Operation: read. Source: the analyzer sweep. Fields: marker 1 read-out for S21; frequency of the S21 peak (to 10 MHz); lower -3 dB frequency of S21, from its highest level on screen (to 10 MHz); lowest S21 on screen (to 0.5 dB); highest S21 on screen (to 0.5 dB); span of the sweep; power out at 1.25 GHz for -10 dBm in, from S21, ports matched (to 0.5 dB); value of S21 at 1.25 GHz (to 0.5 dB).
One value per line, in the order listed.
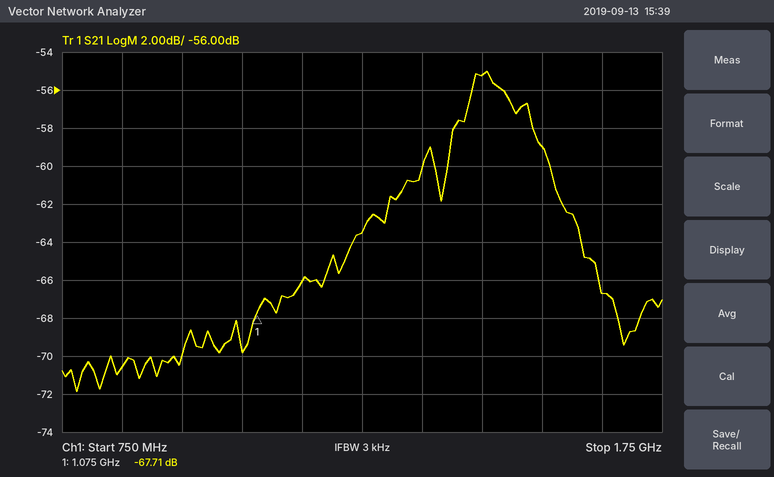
-67.71 dB
1.46 GHz
1.40 GHz
-72.0 dB
-55.0 dB
1 GHz
-73.5 dBm
-63.5 dB
